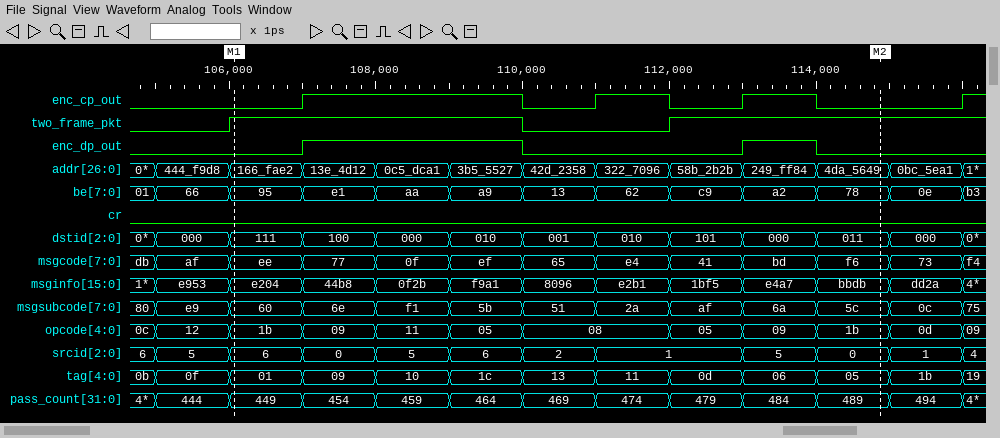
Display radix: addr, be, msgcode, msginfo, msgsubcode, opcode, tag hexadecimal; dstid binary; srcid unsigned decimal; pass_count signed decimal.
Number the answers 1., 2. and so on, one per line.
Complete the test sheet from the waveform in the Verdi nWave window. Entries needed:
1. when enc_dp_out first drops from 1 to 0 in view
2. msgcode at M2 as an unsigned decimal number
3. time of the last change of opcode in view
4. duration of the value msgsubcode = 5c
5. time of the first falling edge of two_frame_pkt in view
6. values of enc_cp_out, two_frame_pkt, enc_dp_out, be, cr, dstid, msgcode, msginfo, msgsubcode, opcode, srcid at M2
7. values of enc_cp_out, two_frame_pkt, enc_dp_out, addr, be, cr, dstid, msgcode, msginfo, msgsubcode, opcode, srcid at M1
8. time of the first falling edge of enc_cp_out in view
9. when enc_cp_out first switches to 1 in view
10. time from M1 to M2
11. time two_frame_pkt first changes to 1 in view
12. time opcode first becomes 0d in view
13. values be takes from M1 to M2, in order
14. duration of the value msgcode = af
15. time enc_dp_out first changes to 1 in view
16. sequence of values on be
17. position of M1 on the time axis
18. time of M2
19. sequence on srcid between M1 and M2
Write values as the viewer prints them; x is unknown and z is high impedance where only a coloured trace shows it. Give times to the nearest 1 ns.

1. 110 ns
2. 246
3. 116 ns
4. 1 ns
5. 110 ns
6. enc_cp_out=0, two_frame_pkt=1, enc_dp_out=0, be=78, cr=0, dstid=011, msgcode=f6, msginfo=bbdb, msgsubcode=5c, opcode=1b, srcid=0
7. enc_cp_out=0, two_frame_pkt=1, enc_dp_out=0, addr=166_fae2, be=95, cr=0, dstid=111, msgcode=ee, msginfo=e204, msgsubcode=60, opcode=1b, srcid=6
8. 110 ns
9. 107 ns
10. 9 ns
11. 106 ns
12. 115 ns
13. 95, e1, aa, a9, 13, 62, c9, a2, 78
14. 1 ns
15. 107 ns
16. 01, 66, 95, e1, aa, a9, 13, 62, c9, a2, 78, 0e, b3
17. 106 ns
18. 115 ns
19. 6, 0, 5, 6, 2, 1, 5, 0
